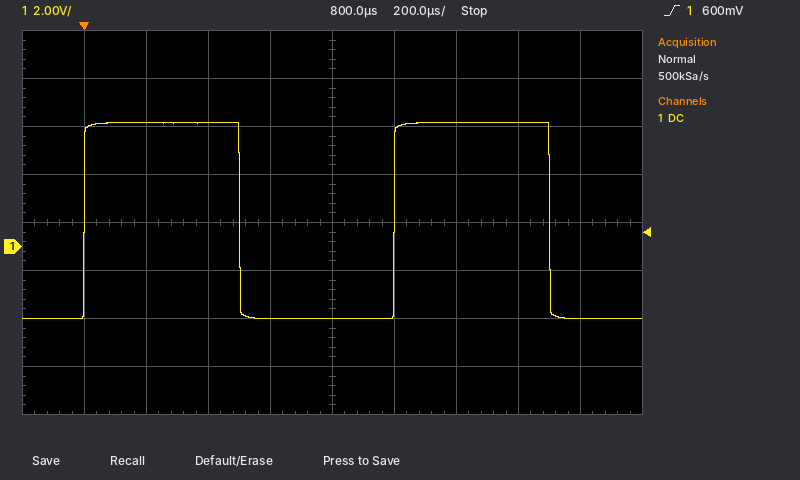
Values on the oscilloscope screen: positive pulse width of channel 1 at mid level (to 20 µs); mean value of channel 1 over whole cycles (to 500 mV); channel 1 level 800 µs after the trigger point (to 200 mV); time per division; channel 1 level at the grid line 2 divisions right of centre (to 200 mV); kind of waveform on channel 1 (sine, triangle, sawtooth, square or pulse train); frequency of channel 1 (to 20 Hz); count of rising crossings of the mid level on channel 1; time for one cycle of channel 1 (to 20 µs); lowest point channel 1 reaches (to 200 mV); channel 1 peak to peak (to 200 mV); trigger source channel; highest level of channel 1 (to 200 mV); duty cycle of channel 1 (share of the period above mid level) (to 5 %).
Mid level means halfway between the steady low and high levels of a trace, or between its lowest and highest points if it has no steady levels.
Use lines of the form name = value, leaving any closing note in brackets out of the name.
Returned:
positive pulse width of channel 1 at mid level = 500 µs
mean value of channel 1 over whole cycles = 1.0 V
channel 1 level 800 µs after the trigger point = -3.0 V
time per division = 200 µs
channel 1 level at the grid line 2 divisions right of centre = 5.2 V
kind of waveform on channel 1 = square
frequency of channel 1 = 1.00 kHz
count of rising crossings of the mid level on channel 1 = 2
time for one cycle of channel 1 = 1.00 ms
lowest point channel 1 reaches = -3.0 V
channel 1 peak to peak = 8.2 V
trigger source channel = channel 1
highest level of channel 1 = 5.2 V
duty cycle of channel 1 (share of the period above mid level) = 50 %
